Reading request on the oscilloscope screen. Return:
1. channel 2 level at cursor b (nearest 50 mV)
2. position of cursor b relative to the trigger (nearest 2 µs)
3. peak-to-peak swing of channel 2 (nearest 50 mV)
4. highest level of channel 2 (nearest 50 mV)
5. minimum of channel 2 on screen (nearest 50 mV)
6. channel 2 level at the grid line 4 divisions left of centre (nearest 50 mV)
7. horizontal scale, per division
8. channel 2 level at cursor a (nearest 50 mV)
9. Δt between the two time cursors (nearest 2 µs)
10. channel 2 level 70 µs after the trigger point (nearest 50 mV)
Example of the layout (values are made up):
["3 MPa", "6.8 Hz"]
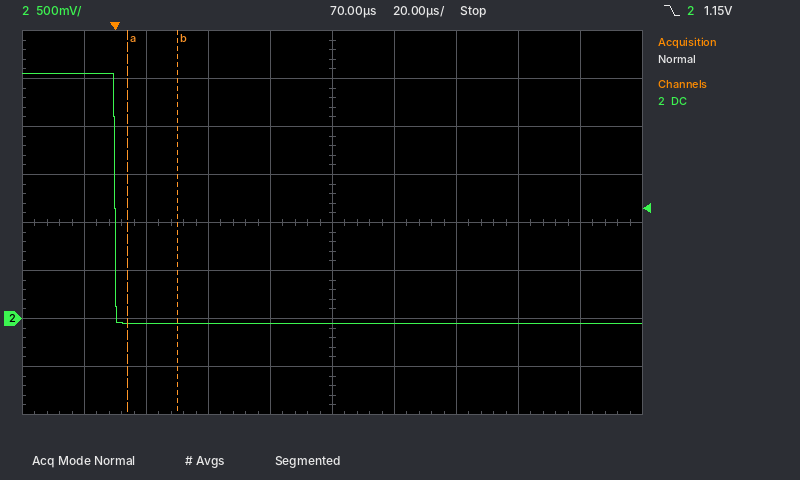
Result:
["-50 mV", "+20 µs", "2.60 V", "2.55 V", "-50 mV", "2.55 V", "20 µs", "-50 mV", "16 µs", "-50 mV"]
